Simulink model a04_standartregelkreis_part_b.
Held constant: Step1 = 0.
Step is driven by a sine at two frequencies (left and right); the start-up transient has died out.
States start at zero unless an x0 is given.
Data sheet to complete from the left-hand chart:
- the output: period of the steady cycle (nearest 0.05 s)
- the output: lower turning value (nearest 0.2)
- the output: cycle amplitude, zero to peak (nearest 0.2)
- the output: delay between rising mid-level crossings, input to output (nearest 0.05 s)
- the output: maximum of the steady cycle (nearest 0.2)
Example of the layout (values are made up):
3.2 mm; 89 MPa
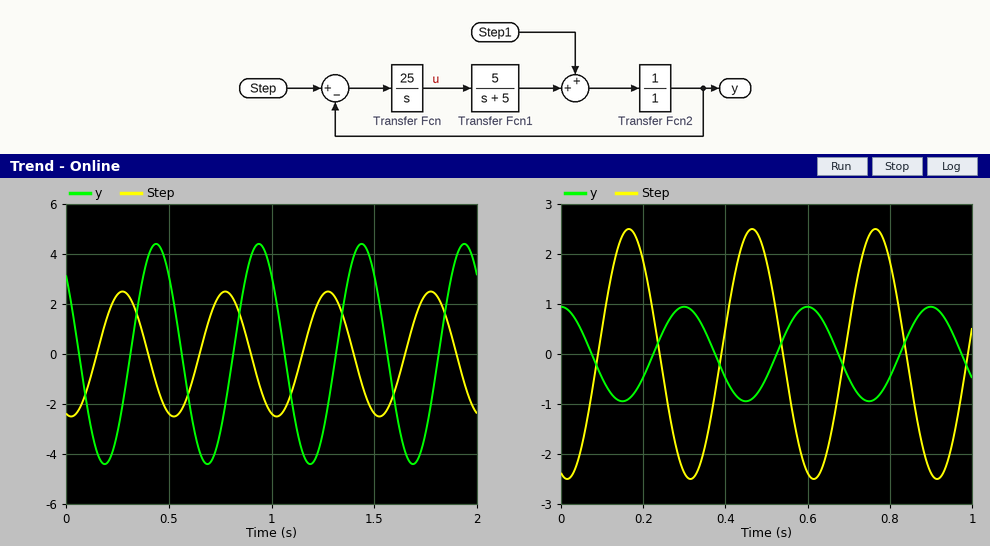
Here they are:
0.50 s; -4.4; 4.4; 0.15 s; 4.4
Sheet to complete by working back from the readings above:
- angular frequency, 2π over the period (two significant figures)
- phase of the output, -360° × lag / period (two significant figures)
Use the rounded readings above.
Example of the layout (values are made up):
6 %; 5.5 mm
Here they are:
13 rad/s; -110°
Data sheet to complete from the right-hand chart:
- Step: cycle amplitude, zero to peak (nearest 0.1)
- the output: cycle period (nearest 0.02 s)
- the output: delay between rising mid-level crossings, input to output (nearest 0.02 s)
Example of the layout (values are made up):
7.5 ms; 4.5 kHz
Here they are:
2.5; 0.30 s; 0.14 s
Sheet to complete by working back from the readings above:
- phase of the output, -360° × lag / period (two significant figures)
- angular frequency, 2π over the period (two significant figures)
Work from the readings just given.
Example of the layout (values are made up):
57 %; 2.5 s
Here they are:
-170°; 21 rad/s
